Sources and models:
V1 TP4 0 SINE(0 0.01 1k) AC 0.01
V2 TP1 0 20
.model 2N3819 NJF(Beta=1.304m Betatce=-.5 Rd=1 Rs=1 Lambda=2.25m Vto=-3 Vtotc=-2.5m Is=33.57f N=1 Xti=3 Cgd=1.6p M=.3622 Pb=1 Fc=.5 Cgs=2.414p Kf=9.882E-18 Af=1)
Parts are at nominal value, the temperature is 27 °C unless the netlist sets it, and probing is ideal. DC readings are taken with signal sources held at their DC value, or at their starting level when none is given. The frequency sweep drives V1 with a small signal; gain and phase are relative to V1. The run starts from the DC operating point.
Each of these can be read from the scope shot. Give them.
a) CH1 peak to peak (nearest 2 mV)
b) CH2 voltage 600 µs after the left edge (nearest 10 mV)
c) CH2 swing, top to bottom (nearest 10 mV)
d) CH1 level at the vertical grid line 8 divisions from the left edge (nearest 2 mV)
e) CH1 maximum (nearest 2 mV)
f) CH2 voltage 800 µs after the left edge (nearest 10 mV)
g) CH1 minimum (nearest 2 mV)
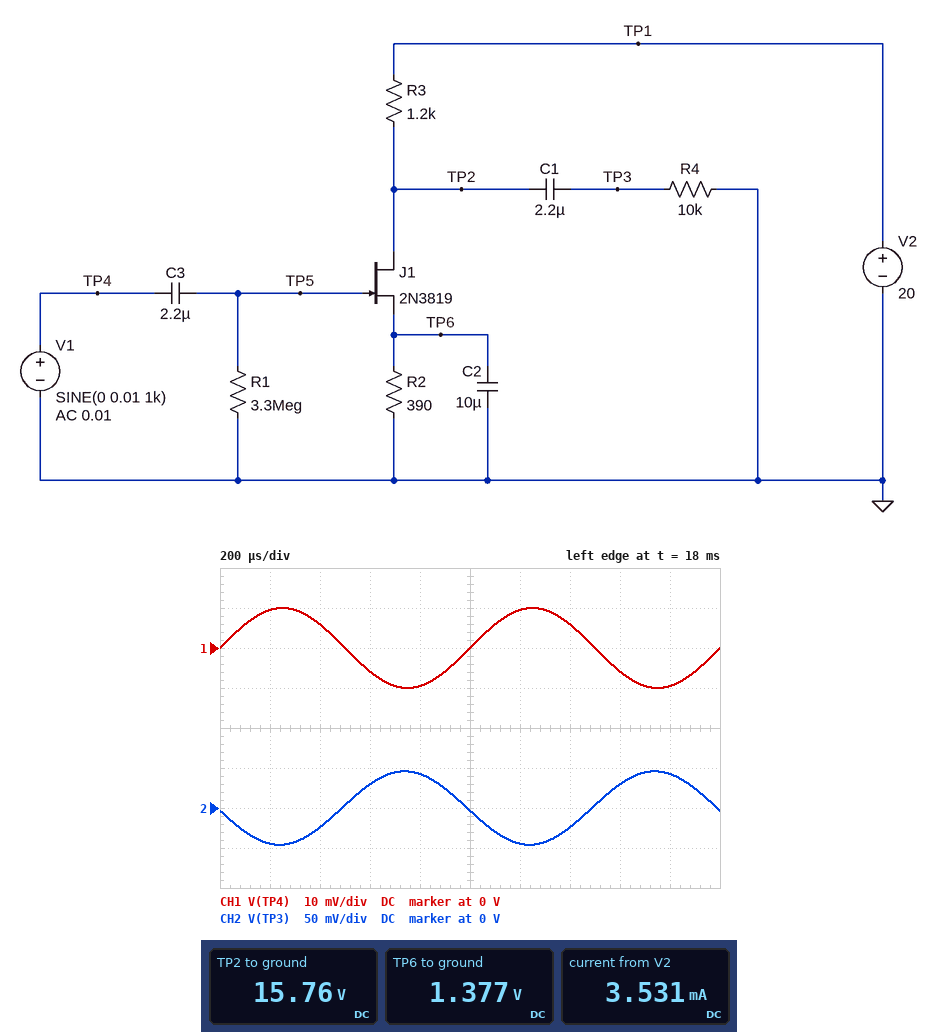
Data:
20 mV
30 mV
90 mV
-6 mV
10 mV
40 mV
-10 mV
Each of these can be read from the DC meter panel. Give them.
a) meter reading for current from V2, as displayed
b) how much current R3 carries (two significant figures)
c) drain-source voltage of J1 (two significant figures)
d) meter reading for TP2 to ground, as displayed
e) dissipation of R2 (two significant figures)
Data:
3.531 mA
3.5 mA
14 V
15.76 V
4.9 mW
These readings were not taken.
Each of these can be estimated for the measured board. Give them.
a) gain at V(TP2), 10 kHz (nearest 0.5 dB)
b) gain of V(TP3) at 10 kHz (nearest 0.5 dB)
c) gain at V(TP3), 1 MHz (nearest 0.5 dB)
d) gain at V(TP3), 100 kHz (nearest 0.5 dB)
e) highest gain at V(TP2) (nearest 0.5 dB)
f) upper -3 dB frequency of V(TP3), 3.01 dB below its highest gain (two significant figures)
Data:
13.5 dB
13.5 dB
13.5 dB
13.5 dB
13.5 dB
400 MHz
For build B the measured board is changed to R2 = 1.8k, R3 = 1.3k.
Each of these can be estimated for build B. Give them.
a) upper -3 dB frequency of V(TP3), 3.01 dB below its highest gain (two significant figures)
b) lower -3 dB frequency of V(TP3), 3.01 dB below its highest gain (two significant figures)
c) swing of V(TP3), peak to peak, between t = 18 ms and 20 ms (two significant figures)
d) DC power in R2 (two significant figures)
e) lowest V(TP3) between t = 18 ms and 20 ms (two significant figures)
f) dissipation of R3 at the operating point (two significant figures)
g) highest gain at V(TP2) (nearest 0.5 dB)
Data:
440 MHz
48 Hz
57 mV
2.4 mW
-29 mV
1.7 mW
9.0 dB
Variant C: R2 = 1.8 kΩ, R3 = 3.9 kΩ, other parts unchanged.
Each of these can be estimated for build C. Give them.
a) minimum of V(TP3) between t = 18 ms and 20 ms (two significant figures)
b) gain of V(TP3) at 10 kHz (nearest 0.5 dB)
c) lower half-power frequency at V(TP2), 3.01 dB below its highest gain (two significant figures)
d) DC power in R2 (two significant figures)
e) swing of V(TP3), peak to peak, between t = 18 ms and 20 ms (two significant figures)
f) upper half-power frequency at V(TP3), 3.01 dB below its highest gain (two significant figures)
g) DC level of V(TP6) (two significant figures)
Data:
-69 mV
17.0 dB
46 Hz
2.4 mW
140 mV
150 MHz
2.1 V
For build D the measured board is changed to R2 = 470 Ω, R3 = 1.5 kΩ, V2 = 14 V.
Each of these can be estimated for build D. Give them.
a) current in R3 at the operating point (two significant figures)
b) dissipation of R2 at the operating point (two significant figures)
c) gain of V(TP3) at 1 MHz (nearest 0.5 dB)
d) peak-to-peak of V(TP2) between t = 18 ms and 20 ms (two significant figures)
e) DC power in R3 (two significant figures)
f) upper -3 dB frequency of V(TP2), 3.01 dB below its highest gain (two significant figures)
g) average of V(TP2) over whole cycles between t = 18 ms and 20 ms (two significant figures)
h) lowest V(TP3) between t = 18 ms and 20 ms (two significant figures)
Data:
3.1 mA
4.6 mW
14.5 dB
100 mV
15 mW
260 MHz
9.3 V
-52 mV
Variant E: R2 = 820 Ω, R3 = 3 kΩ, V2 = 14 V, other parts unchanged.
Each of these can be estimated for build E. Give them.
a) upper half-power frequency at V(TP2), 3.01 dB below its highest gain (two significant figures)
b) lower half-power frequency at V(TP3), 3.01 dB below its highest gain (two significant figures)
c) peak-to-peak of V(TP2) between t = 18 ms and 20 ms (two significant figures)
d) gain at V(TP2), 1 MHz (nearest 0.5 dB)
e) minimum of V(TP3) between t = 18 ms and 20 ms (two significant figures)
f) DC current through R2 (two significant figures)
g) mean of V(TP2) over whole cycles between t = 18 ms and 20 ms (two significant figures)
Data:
130 MHz
67 Hz
150 mV
17.5 dB
-76 mV
2.1 mA
7.7 V
